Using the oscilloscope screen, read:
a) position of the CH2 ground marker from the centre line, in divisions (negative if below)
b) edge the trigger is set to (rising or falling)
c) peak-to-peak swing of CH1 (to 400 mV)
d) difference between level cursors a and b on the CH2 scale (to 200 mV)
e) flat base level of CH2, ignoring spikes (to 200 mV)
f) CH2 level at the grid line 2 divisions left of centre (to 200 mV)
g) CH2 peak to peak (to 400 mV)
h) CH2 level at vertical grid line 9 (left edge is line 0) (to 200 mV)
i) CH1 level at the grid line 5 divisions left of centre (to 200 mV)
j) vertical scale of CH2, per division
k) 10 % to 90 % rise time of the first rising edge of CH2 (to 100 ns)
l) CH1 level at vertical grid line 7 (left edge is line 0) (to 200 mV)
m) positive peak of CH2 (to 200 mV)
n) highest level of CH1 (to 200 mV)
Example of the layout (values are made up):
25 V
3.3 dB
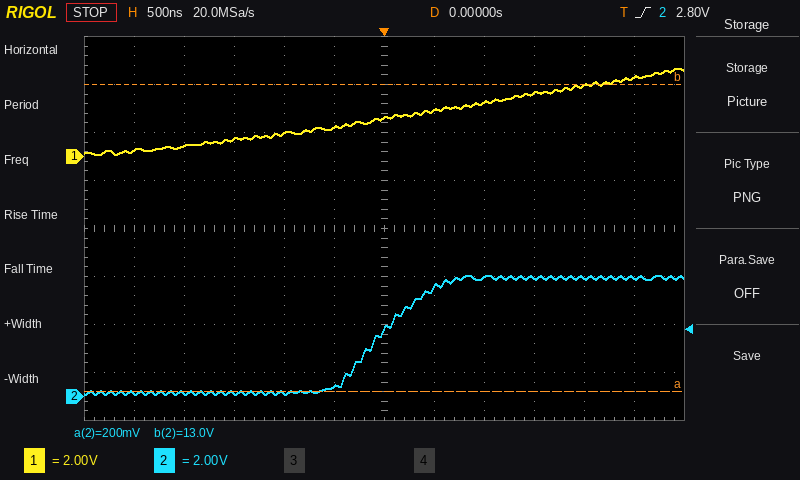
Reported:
-3.5 div
rising
3.6 V
12.8 V
200 mV
200 mV
4.8 V
5.0 V
200 mV
2 V
900 ns
2.0 V
5.0 V
3.6 V
